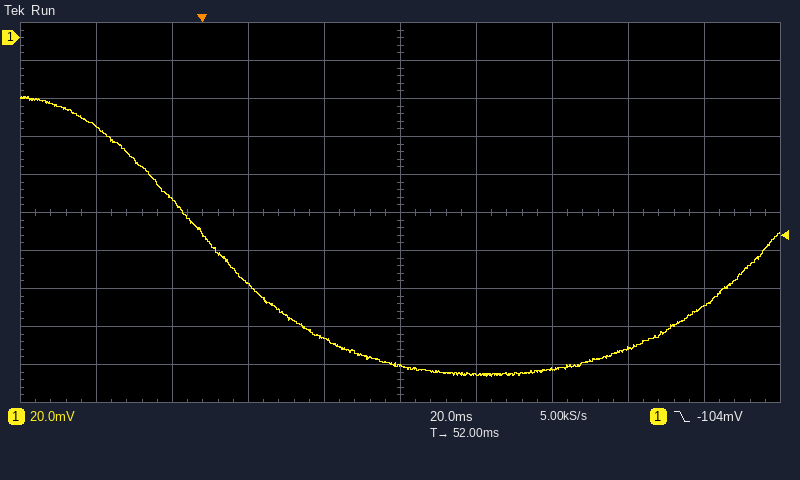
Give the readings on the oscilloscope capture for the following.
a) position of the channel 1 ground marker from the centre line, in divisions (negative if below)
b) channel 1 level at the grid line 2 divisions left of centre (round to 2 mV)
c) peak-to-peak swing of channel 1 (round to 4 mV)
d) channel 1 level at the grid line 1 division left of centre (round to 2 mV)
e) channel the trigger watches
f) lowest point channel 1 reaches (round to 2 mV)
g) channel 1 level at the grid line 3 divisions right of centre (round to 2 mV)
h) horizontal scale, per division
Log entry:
+4.6 div
-130 mV
148 mV
-158 mV
channel 1
-178 mV
-164 mV
20 ms
